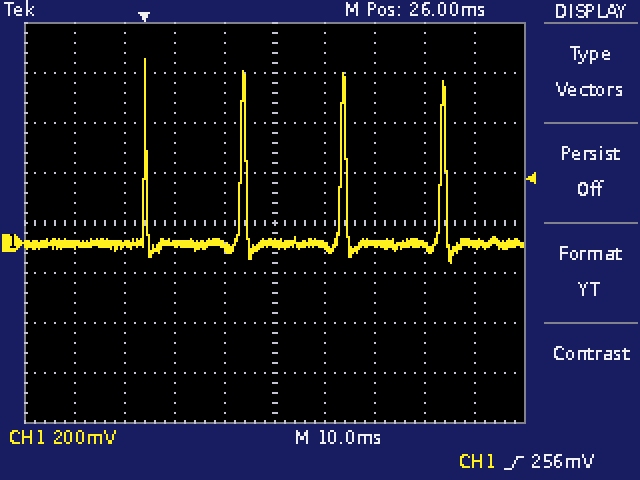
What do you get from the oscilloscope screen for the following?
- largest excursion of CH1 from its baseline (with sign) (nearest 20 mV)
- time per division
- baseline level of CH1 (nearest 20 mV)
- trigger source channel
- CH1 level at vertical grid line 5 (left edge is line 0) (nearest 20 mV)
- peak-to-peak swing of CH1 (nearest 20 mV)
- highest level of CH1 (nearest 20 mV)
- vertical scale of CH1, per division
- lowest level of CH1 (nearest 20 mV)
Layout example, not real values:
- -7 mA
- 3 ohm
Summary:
- +740 mV
- 10 ms
- 0 mV
- CH1
- 0 mV
- 820 mV
- 740 mV
- 200 mV
- -80 mV
